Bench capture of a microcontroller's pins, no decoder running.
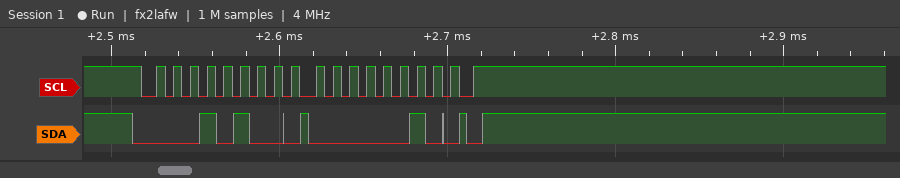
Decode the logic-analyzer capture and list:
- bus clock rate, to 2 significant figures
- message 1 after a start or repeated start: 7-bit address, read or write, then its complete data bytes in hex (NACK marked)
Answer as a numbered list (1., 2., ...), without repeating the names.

1. 100 kHz
2. 0x0A write: 02
